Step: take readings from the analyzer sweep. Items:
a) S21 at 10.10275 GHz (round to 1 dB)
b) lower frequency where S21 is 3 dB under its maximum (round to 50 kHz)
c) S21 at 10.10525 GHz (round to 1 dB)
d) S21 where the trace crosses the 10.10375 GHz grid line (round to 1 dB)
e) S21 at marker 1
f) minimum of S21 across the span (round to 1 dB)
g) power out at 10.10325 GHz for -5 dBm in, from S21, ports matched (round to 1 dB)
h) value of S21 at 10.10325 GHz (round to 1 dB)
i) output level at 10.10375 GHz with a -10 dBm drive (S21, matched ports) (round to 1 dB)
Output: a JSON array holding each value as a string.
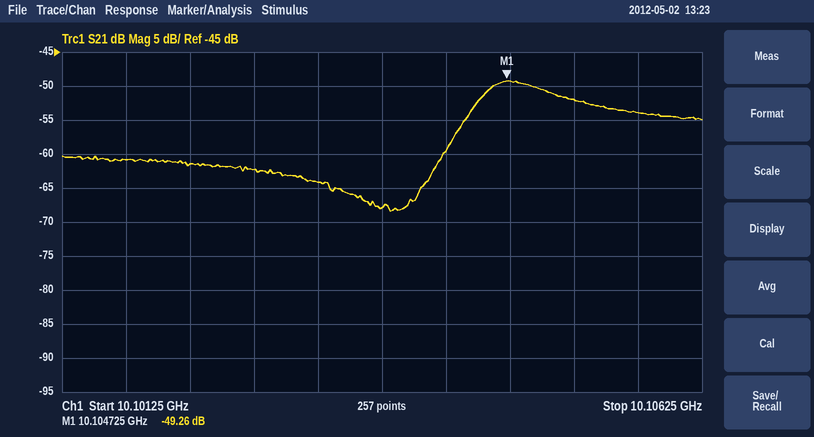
["-62 dB", "10.10450 GHz", "-52 dB", "-68 dB", "-49.26 dB", "-68 dB", "-69 dBm", "-64 dB", "-78 dBm"]
